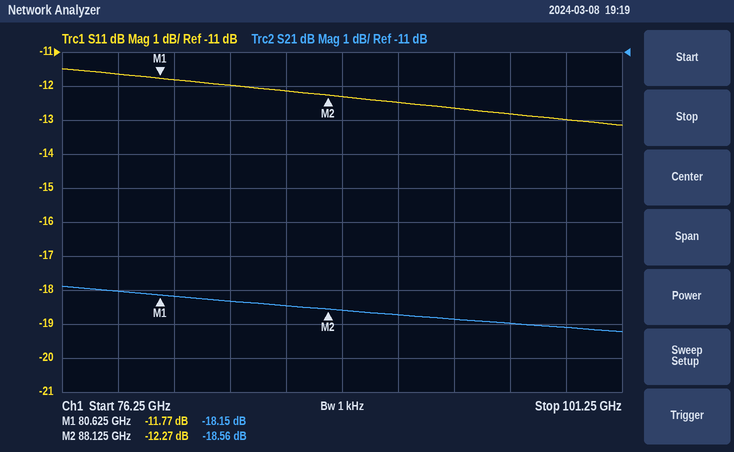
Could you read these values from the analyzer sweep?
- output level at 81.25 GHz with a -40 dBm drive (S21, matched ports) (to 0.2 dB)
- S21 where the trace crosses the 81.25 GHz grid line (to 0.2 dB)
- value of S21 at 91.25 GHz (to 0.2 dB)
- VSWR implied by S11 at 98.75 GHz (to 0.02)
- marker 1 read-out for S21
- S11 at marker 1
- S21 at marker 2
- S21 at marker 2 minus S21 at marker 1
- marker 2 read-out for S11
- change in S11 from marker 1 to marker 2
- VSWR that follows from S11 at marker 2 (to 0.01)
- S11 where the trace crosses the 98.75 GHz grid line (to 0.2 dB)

-58.2 dBm
-18.2 dB
-18.8 dB
1.58
-18.15 dB
-11.77 dB
-18.56 dB
-0.41 dB
-12.27 dB
-0.50 dB
1.64
-13.0 dB
